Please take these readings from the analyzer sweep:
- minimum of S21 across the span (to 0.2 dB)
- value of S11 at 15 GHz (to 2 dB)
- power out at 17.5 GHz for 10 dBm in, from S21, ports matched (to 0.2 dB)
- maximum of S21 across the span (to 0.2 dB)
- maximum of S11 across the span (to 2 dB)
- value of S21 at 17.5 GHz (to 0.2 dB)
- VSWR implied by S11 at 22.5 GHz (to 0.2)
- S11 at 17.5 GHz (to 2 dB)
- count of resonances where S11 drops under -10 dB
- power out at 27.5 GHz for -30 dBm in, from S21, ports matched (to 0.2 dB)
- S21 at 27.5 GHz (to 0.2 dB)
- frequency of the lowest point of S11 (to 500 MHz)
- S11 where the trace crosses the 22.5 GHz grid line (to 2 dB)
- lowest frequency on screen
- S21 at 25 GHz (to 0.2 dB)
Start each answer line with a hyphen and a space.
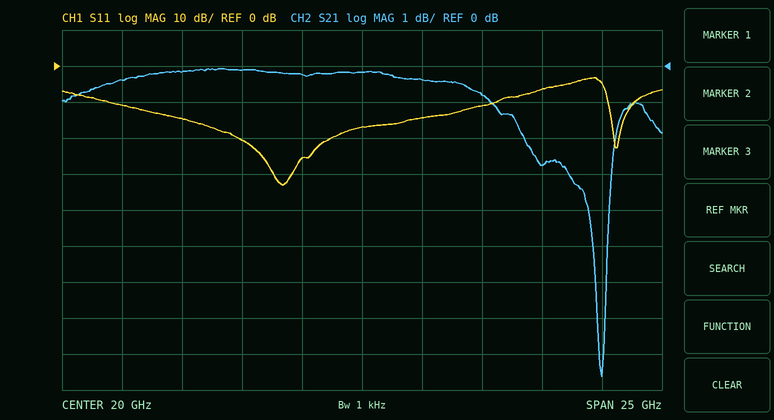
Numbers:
- -8.6 dB
- -20 dB
- 9.8 dBm
- 0.0 dB
- -4 dB
- -0.2 dB
- 1.4
- -26 dB
- 2
- -32.8 dBm
- -2.8 dB
- 16.5 GHz
- -14 dB
- 7.5 GHz
- -0.8 dB
